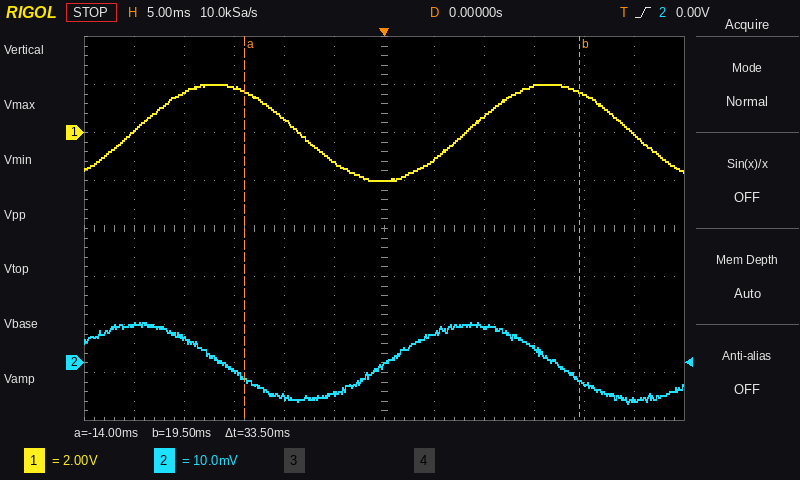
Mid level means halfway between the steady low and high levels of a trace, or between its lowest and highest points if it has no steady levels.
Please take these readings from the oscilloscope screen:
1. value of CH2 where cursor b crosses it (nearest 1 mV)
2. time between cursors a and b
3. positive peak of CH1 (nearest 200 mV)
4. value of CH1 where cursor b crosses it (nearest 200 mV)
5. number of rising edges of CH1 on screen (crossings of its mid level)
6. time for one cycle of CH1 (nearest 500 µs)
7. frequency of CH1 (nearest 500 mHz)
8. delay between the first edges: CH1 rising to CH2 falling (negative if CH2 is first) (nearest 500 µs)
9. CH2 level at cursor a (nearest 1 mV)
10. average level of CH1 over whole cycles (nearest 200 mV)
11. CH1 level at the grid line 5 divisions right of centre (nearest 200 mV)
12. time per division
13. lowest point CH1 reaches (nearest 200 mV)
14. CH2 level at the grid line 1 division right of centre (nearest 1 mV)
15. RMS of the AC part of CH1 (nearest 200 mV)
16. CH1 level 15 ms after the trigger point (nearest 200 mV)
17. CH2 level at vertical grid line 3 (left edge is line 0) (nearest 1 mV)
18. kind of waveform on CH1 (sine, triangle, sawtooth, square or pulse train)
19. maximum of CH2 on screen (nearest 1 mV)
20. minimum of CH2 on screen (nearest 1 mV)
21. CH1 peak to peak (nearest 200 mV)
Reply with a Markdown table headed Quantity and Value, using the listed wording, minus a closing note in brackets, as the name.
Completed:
| Quantity | Value |
|---|---|
| value of CH2 where cursor b crosses it | -3 mV |
| time between cursors a and b | 33.5 ms |
| positive peak of CH1 | 2.0 V |
| value of CH1 where cursor b crosses it | 1.6 V |
| number of rising edges of CH1 on screen | 2 |
| time for one cycle of CH1 | 33.5 ms |
| frequency of CH1 | 30.0 Hz |
| delay between the first edges: CH1 rising to CH2 falling (negative if CH2 is first) | +9.0 ms |
| CH2 level at cursor a | -3 mV |
| average level of CH1 over whole cycles | 0.0 V |
| CH1 level at the grid line 5 divisions right of centre | 0.0 V |
| time per division | 5 ms |
| lowest point CH1 reaches | -2.0 V |
| CH2 level at the grid line 1 division right of centre | 6 mV |
| RMS of the AC part of CH1 | 1.4 V |
| CH1 level 15 ms after the trigger point | 2.0 V |
| CH2 level at vertical grid line 3 (left edge is line 0) | -2 mV |
| kind of waveform on CH1 | sine |
| maximum of CH2 on screen | 8 mV |
| minimum of CH2 on screen | -8 mV |
| CH1 peak to peak | 4.0 V |
